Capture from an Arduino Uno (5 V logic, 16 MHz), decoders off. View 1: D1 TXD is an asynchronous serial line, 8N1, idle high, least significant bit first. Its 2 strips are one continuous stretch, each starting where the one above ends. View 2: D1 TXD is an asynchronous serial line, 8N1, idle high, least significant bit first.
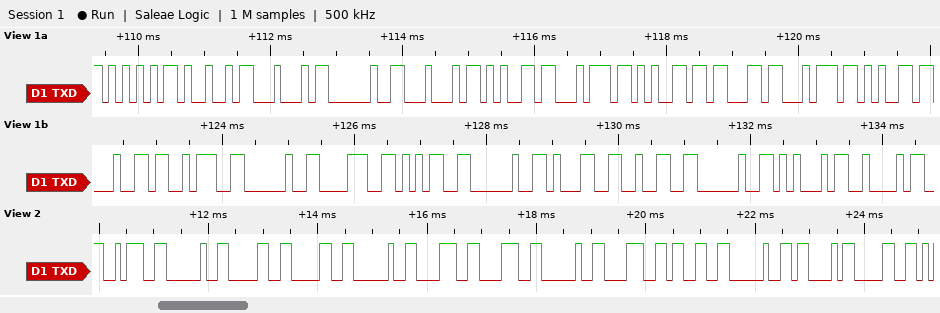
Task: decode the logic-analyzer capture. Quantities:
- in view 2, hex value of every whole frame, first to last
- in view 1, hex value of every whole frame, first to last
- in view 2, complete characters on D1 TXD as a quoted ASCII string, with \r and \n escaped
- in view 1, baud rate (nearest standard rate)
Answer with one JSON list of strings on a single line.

["3A 20 30 30 20 38 38 20 38 33 20 43 30", "55 49 44 20 44 65 74 65 63 74 65 64 3A 20 38 35 20 31 32 20 45 42", "\": 00 88 83 C0\"", "9600 baud"]
